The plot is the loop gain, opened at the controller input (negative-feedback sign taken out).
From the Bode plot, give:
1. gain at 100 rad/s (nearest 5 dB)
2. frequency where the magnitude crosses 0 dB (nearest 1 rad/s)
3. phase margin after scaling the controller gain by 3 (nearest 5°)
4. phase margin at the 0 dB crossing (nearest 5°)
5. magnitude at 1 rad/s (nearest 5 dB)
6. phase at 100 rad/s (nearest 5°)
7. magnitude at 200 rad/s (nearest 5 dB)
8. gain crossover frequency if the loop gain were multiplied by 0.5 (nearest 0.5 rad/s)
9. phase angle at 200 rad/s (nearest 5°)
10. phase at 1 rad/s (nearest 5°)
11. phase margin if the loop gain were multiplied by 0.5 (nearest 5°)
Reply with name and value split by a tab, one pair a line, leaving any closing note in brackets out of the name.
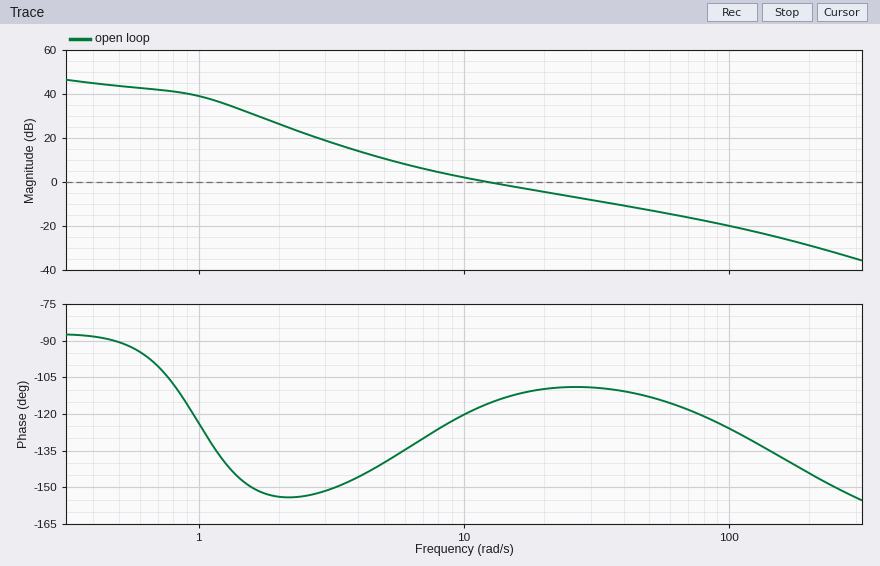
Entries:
gain at 100 rad/s	-20 dB
frequency where the magnitude crosses 0 dB	12 rad/s
phase margin after scaling the controller gain by 3	70°
phase margin at the 0 dB crossing	65°
magnitude at 1 rad/s	40 dB
phase at 100 rad/s	-125°
magnitude at 200 rad/s	-30 dB
gain crossover frequency if the loop gain were multiplied by 0.5	7.0 rad/s
phase angle at 200 rad/s	-145°
phase at 1 rad/s	-125°
phase margin if the loop gain were multiplied by 0.5	50°
